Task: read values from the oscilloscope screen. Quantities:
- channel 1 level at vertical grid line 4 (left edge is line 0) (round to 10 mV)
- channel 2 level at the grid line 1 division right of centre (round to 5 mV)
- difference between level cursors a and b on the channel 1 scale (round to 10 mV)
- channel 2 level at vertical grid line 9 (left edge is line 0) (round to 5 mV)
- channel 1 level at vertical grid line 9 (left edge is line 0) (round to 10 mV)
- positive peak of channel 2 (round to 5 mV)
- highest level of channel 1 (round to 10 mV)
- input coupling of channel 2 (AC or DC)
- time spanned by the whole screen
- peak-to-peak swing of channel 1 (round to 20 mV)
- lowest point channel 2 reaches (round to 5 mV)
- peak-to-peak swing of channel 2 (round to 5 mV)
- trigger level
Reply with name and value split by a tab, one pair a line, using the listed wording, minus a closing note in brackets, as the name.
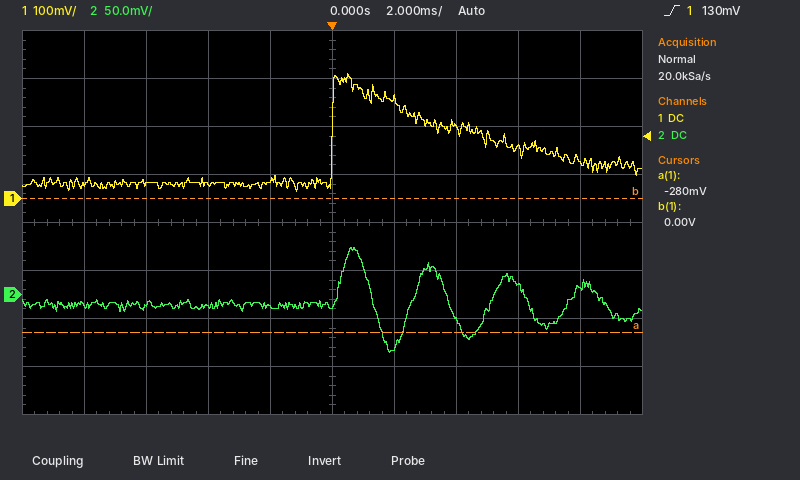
channel 1 level at vertical grid line 4 (left edge is line 0)	40 mV
channel 2 level at the grid line 1 division right of centre	-55 mV
difference between level cursors a and b on the channel 1 scale	280 mV
channel 2 level at vertical grid line 9 (left edge is line 0)	10 mV
channel 1 level at vertical grid line 9 (left edge is line 0)	80 mV
positive peak of channel 2	50 mV
highest level of channel 1	260 mV
input coupling of channel 2	DC
time spanned by the whole screen	20 ms
peak-to-peak swing of channel 1	240 mV
lowest point channel 2 reaches	-60 mV
peak-to-peak swing of channel 2	110 mV
trigger level	130 mV
